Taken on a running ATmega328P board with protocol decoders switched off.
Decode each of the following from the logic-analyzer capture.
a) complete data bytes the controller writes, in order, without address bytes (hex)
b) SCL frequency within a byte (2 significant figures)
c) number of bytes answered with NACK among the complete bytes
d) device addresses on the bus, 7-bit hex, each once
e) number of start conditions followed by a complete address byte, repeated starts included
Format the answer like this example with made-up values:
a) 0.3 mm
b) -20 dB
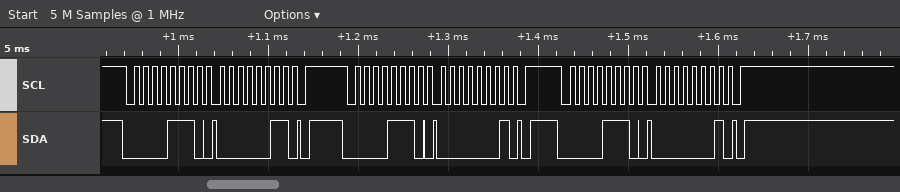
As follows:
a) 03 01 01
b) 100 kHz
c) 0
d) 0x07
e) 3
